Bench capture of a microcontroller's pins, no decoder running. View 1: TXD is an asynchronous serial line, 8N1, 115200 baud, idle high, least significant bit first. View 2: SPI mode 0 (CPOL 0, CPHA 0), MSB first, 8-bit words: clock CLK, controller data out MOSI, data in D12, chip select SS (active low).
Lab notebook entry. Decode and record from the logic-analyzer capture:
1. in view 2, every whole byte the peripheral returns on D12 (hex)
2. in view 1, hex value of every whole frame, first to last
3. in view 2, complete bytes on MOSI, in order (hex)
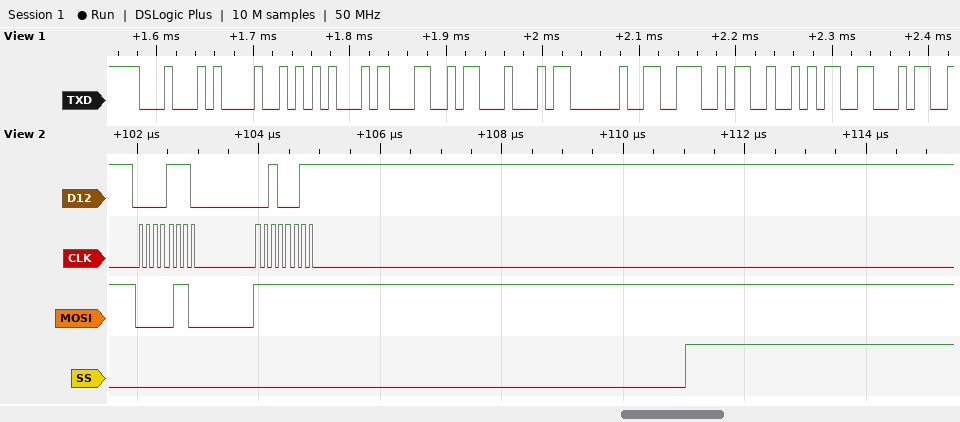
0x0E 0x23
0x44 0x48 0x45 0x4C 0x44 0x20 0x4E 0x52 0x46
0x06 0xFF
